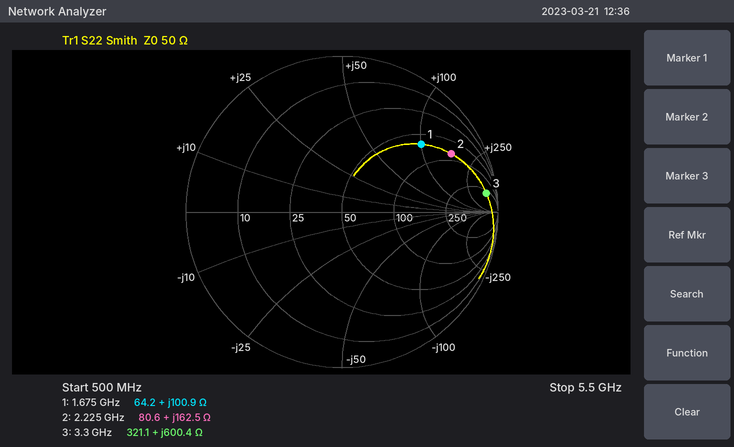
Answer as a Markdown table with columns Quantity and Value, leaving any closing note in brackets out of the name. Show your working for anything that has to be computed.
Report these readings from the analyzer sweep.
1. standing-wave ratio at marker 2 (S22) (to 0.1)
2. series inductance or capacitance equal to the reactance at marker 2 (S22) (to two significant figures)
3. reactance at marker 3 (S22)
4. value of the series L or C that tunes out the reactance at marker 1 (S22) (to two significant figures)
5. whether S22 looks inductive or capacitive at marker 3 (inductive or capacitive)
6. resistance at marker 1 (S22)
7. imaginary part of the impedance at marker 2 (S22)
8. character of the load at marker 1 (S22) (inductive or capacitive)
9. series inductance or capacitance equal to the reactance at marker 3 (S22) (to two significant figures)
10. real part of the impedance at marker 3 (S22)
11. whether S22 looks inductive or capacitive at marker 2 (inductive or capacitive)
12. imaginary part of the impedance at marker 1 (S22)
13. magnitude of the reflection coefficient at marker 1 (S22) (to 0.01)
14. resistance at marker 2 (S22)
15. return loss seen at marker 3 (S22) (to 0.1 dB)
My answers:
| Quantity | Value |
|---|---|
| standing-wave ratio at marker 2 (S22) | 8.7 |
| series inductance or capacitance equal to the reactance at marker 2 (S22) | L = 162.5 Ω/(2π × 2.225 GHz) ≈ 12 nH |
| reactance at marker 3 | +600.4 Ω |
| value of the series L or C that tunes out the reactance at marker 1 (S22) | C = 1/(2π × 1.675 GHz × 100.9 Ω) ≈ 942 fF, so 940 fF to two significant figures |
| whether S22 looks inductive or capacitive at marker 3 | inductive |
| resistance at marker 1 | 64.2 Ω |
| imaginary part of the impedance at marker 2 | +162.5 Ω |
| character of the load at marker 1 (S22) | inductive |
| series inductance or capacitance equal to the reactance at marker 3 (S22) | L = 600.4 Ω/(2π × 3.3 GHz) ≈ 29 nH |
| real part of the impedance at marker 3 | 321.1 Ω |
| whether S22 looks inductive or capacitive at marker 2 | inductive |
| imaginary part of the impedance at marker 1 | +100.9 Ω |
| magnitude of the reflection coefficient at marker 1 (S22) | 0.67 |
| resistance at marker 2 | 80.6 Ω |
| return loss seen at marker 3 (S22) | 0.6 dB |
